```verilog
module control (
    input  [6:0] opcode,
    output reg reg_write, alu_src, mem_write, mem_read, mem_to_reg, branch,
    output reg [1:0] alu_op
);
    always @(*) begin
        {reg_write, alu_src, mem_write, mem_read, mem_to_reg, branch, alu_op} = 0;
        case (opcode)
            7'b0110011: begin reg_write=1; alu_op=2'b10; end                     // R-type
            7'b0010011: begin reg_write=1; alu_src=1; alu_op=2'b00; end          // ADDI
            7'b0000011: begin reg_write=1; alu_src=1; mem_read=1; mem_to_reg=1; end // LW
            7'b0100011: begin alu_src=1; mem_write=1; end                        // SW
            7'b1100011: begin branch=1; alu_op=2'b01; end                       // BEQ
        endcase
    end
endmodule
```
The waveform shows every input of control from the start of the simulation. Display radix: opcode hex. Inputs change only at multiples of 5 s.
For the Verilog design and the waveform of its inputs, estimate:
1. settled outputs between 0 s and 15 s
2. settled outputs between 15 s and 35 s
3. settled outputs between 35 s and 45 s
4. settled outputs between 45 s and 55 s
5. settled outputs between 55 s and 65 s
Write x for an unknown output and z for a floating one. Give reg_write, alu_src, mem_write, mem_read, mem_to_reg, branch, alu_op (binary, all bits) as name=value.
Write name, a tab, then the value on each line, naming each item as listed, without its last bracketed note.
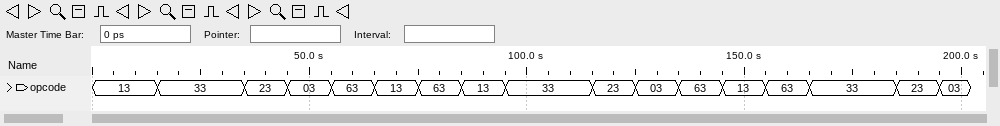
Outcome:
settled outputs between 0 s and 15 s	reg_write=1, alu_src=1, mem_write=0, mem_read=0, mem_to_reg=0, branch=0, alu_op=00
settled outputs between 15 s and 35 s	reg_write=1, alu_src=0, mem_write=0, mem_read=0, mem_to_reg=0, branch=0, alu_op=10
settled outputs between 35 s and 45 s	reg_write=0, alu_src=1, mem_write=1, mem_read=0, mem_to_reg=0, branch=0, alu_op=00
settled outputs between 45 s and 55 s	reg_write=1, alu_src=1, mem_write=0, mem_read=1, mem_to_reg=1, branch=0, alu_op=00
settled outputs between 55 s and 65 s	reg_write=0, alu_src=0, mem_write=0, mem_read=0, mem_to_reg=0, branch=1, alu_op=01
